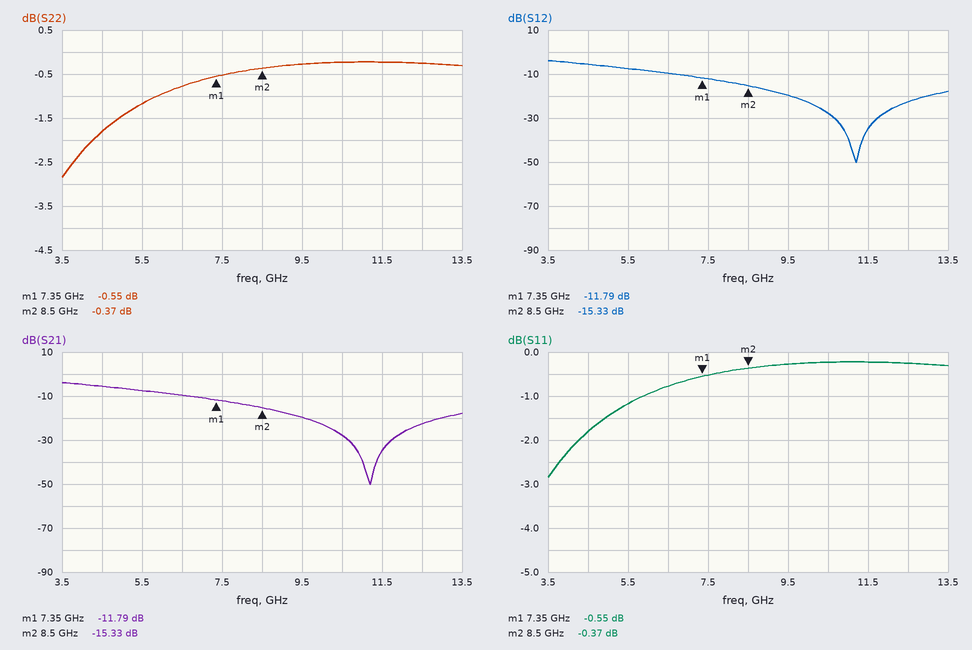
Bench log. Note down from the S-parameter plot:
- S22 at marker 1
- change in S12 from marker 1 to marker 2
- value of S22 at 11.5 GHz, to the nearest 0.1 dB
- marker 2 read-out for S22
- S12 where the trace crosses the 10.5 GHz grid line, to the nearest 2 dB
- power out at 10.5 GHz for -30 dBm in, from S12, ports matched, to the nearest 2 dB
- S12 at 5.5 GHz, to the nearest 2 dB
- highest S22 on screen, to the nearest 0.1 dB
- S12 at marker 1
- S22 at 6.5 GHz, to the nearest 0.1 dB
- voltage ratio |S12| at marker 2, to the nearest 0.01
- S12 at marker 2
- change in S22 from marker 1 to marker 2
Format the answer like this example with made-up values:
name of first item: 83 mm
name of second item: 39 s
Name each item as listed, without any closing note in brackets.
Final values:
S22 at marker 1: -0.55 dB
change in S12 from marker 1 to marker 2: -3.54 dB
value of S22 at 11.5 GHz, to the nearest 0.1 dB: -0.2 dB
marker 2 read-out for S22: -0.37 dB
S12 where the trace crosses the 10.5 GHz grid line, to the nearest 2 dB: -28 dB
power out at 10.5 GHz for -30 dBm in, from S12, ports matched, to the nearest 2 dB: -58 dBm
S12 at 5.5 GHz, to the nearest 2 dB: -8 dB
highest S22 on screen, to the nearest 0.1 dB: -0.2 dB
S12 at marker 1: -11.79 dB
S22 at 6.5 GHz, to the nearest 0.1 dB: -0.8 dB
voltage ratio |S12| at marker 2, to the nearest 0.01: 0.17
S12 at marker 2: -15.33 dB
change in S22 from marker 1 to marker 2: 0.18 dB
